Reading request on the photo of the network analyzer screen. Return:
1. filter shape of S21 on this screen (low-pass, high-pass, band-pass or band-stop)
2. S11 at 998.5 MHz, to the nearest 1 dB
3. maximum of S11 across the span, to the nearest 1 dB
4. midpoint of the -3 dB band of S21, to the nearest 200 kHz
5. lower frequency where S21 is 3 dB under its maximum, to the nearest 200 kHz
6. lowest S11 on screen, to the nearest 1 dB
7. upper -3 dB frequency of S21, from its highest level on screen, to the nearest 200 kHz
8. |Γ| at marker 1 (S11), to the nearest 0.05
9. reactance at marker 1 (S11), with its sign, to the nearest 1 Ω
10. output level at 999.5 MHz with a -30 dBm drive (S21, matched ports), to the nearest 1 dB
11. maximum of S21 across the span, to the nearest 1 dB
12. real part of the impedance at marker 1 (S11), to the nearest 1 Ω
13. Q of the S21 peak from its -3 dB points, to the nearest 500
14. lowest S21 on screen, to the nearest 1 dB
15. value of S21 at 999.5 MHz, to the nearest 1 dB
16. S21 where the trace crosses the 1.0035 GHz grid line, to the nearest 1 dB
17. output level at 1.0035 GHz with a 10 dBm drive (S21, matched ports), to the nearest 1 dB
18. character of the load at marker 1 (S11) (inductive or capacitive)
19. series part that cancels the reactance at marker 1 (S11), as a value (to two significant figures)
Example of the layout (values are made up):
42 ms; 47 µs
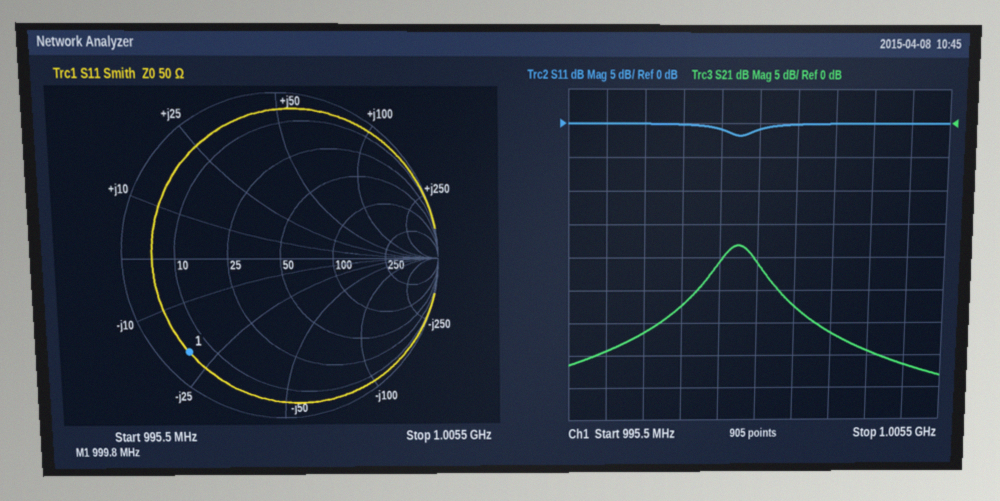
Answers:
band-pass; 0 dB; 0 dB; 1.0000 GHz; 999.4 MHz; -2 dB; 1.0006 GHz; 0.85; -20 Ω; -51 dBm; -18 dB; 5 Ω; 1000; -38 dB; -21 dB; -34 dB; -24 dBm; capacitive; 3.2 nH
